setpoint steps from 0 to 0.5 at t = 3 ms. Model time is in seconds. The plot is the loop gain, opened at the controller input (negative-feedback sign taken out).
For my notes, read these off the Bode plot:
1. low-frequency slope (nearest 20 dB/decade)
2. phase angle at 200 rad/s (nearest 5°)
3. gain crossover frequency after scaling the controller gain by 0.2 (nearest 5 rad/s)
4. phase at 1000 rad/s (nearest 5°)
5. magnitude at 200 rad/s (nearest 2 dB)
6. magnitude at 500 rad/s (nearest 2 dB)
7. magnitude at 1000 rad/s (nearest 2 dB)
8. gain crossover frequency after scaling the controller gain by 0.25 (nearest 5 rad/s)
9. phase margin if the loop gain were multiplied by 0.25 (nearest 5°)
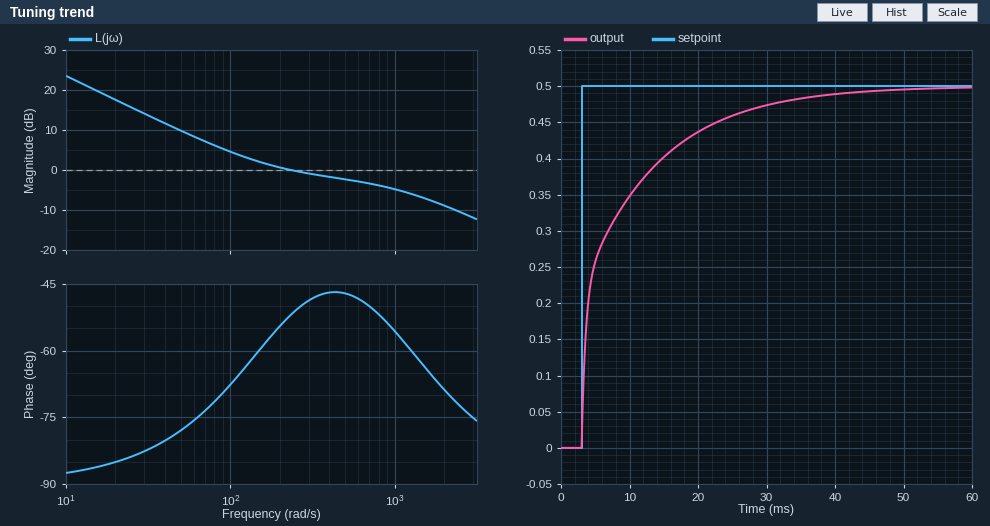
-20 dB/decade
-55°
30 rad/s
-55°
0 dB
-2 dB
-4 dB
40 rad/s
100°
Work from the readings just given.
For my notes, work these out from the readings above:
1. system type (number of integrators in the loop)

1
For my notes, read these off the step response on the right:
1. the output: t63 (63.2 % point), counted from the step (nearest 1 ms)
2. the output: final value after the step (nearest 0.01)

5 ms
0.50
